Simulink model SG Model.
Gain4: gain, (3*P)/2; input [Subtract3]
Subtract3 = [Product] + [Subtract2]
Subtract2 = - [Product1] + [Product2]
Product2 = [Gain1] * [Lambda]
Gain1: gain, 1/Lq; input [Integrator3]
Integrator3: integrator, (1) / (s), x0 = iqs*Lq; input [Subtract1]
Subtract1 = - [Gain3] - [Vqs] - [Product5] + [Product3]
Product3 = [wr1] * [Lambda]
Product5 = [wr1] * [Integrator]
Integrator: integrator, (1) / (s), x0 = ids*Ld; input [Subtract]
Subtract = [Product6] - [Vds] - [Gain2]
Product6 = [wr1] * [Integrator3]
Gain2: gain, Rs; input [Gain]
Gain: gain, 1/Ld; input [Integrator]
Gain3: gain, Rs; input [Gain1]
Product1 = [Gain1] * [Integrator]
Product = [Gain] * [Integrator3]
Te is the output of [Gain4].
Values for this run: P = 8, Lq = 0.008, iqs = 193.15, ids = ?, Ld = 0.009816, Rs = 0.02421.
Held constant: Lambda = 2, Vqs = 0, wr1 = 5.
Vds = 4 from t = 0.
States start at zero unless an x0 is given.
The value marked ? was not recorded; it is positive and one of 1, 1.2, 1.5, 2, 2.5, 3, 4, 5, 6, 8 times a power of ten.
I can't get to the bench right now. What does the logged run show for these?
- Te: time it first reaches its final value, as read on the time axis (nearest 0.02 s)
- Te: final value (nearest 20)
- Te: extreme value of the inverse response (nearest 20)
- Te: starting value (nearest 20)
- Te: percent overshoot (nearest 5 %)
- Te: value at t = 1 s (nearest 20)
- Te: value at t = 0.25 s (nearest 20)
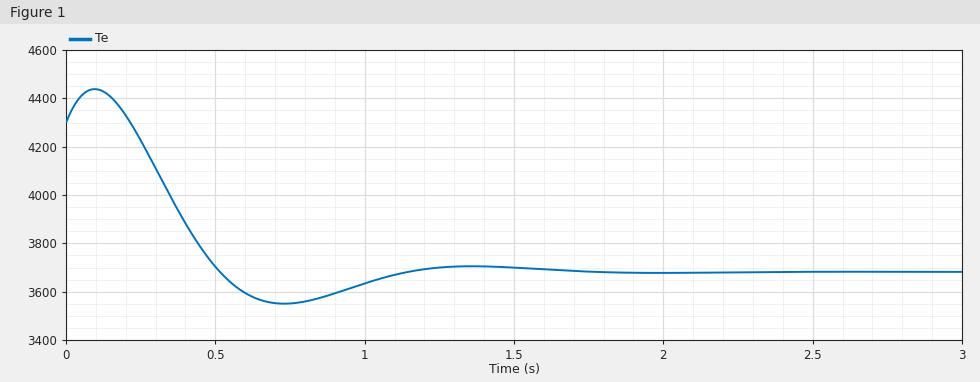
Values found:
0.52 s
3680
4440
4300
20 %
3640
4220
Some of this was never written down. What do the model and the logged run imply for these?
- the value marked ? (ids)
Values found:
80
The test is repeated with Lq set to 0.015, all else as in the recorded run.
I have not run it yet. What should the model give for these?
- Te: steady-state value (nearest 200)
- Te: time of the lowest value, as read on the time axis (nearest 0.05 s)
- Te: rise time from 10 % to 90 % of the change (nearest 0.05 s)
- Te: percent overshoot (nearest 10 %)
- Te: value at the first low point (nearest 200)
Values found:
3400
0.70 s
0.15 s
40 %
2600
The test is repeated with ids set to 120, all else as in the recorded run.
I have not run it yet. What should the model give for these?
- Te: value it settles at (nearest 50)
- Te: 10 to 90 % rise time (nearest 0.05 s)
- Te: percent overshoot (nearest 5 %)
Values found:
3700
0.20 s
25 %
